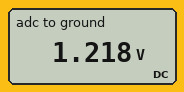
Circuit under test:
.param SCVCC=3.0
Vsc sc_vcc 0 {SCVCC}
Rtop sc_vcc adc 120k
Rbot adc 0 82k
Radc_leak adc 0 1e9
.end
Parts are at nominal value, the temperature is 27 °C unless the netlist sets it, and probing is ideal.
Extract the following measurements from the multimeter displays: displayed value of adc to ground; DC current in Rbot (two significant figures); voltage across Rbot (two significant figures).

1.218 V
15 µA
1.2 V
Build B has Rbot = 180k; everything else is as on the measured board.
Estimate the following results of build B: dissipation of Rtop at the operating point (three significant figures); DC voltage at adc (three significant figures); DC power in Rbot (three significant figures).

12.0 µW
1.80 V
18.0 µW
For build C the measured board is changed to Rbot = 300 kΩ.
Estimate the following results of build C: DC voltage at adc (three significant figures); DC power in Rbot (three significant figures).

2.14 V
15.3 µW
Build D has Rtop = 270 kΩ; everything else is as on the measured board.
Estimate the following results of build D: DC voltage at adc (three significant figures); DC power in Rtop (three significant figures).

699 mV
19.6 µW
